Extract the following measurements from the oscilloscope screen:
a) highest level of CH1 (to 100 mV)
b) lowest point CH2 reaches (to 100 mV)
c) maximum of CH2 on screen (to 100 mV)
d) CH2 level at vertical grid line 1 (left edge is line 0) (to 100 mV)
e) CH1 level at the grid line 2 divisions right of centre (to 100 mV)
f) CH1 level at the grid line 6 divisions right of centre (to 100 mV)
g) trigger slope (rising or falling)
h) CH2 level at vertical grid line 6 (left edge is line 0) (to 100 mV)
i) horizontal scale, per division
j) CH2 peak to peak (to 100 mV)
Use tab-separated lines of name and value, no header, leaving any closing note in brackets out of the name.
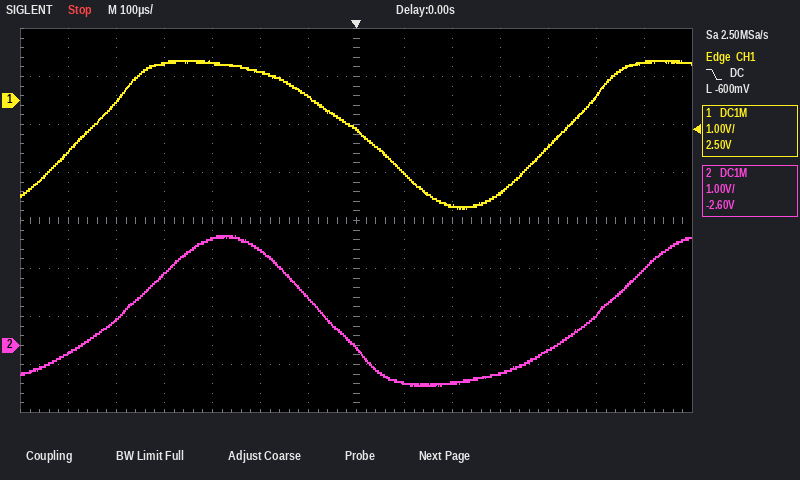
highest level of CH1	800 mV
lowest point CH2 reaches	-800 mV
maximum of CH2 on screen	2.3 V
CH2 level at vertical grid line 1 (left edge is line 0)	-200 mV
CH1 level at the grid line 2 divisions right of centre	-2.2 V
CH1 level at the grid line 6 divisions right of centre	800 mV
trigger slope	falling
CH2 level at vertical grid line 6 (left edge is line 0)	1.0 V
horizontal scale, per division	100 µs
CH2 peak to peak	3.1 V
